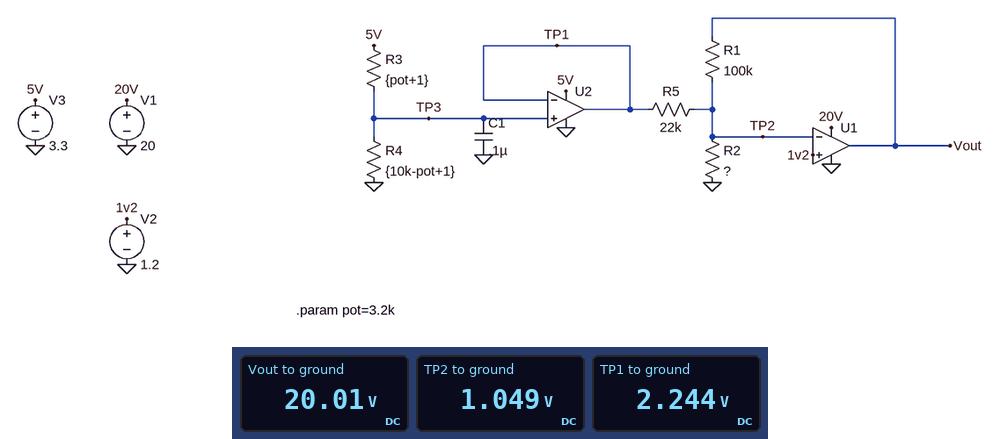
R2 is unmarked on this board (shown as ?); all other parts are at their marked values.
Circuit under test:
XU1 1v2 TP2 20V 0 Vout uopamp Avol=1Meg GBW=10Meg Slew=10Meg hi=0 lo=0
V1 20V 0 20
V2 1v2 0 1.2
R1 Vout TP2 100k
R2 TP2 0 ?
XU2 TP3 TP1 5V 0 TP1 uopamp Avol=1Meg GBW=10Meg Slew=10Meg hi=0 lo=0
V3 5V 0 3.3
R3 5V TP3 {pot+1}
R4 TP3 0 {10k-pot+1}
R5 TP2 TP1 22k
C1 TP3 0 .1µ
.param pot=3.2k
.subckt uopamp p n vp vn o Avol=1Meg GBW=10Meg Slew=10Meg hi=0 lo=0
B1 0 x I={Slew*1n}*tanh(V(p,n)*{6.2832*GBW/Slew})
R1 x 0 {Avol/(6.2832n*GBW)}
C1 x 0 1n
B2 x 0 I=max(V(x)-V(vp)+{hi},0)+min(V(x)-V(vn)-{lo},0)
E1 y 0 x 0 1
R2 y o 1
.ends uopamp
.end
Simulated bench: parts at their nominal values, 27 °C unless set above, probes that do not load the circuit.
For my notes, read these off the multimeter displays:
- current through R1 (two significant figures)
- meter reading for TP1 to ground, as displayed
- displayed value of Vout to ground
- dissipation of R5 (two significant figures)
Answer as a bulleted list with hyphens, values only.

- 190 µA
- 2.244 V
- 20.01 V
- 65 µW
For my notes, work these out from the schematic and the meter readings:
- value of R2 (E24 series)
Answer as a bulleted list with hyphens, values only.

- 4.3 kΩ
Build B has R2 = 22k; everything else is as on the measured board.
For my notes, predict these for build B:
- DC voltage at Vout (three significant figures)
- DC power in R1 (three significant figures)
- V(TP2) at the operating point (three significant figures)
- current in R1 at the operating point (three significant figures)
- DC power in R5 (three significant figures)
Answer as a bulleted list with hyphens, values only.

- 1.91 V
- 5.04 µW
- 1.20 V
- 7.10 µA
- 49.5 µW
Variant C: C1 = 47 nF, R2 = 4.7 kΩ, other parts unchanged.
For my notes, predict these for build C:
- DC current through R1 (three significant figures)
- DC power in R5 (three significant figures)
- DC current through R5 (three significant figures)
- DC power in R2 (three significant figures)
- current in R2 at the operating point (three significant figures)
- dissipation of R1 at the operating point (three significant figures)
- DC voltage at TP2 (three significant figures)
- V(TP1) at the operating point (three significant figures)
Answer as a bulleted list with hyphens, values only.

- 189 µA
- 56.8 µW
- 50.8 µA
- 270 µW
- 240 µA
- 3.56 mW
- 1.13 V
- 2.24 V
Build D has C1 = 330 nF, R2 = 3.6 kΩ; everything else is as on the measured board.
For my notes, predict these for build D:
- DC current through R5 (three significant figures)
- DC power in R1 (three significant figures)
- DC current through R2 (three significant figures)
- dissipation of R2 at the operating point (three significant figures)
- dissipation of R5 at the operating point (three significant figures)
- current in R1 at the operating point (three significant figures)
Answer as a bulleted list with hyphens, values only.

- 60.8 µA
- 3.65 mW
- 252 µA
- 228 µW
- 81.3 µW
- 191 µA
